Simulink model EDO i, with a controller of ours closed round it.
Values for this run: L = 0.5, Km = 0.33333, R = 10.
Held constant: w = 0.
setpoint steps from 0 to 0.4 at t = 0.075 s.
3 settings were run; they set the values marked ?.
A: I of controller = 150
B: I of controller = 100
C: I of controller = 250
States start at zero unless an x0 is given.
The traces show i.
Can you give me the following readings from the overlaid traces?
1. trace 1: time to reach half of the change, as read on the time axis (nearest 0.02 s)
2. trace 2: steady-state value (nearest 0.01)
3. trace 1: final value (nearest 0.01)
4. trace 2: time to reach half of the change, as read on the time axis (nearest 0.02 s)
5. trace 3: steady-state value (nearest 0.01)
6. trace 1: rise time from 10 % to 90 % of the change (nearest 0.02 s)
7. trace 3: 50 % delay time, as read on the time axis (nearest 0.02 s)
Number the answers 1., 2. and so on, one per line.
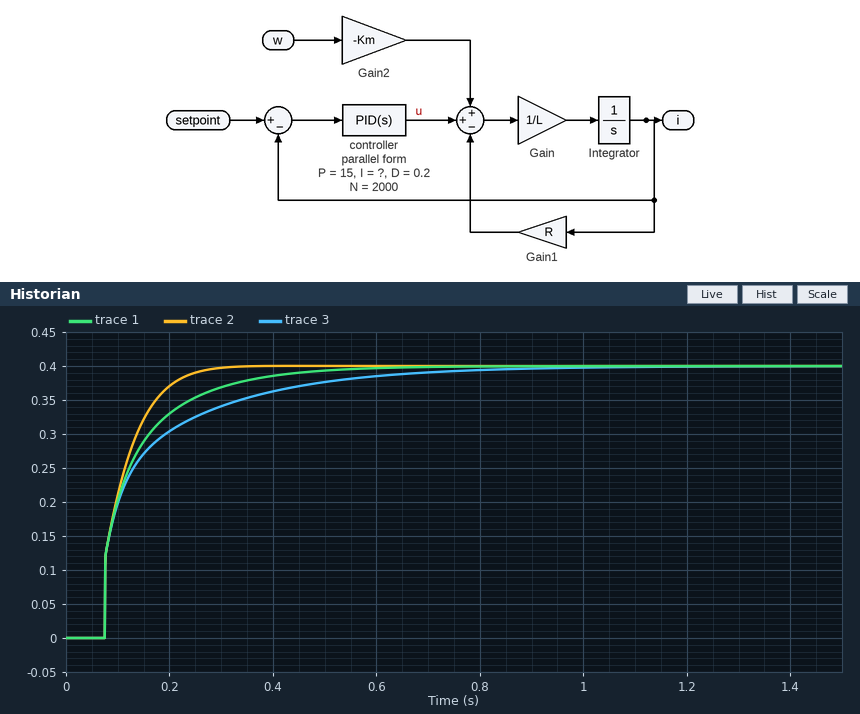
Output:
1. 0.10 s
2. 0.40
3. 0.40
4. 0.10 s
5. 0.40
6. 0.20 s
7. 0.10 s
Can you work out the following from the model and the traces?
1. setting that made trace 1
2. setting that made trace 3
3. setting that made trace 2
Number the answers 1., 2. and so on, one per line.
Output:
1. A
2. B
3. C
